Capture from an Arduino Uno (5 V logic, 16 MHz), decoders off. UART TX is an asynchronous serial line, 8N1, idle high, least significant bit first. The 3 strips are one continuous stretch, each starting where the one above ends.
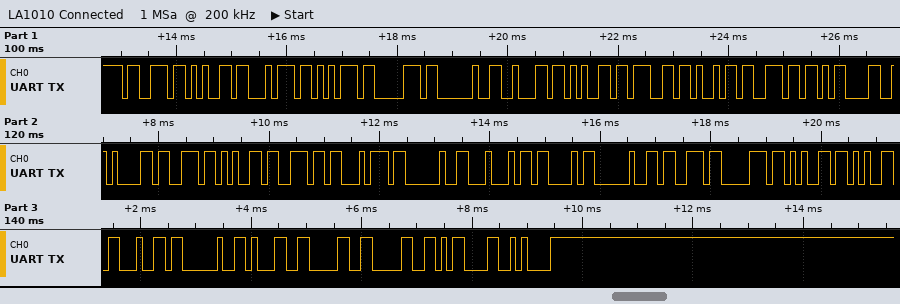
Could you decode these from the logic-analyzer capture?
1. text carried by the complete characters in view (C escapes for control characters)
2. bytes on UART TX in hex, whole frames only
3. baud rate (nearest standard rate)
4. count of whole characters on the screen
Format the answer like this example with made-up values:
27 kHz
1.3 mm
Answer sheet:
"setup begin\r\nsent DC speed 100\r\n"
73 65 74 75 70 20 62 65 67 69 6E 0D 0A 73 65 6E 74 20 44 43 20 73 70 65 65 64 20 31 30 30 0D 0A
9600 baud
32
